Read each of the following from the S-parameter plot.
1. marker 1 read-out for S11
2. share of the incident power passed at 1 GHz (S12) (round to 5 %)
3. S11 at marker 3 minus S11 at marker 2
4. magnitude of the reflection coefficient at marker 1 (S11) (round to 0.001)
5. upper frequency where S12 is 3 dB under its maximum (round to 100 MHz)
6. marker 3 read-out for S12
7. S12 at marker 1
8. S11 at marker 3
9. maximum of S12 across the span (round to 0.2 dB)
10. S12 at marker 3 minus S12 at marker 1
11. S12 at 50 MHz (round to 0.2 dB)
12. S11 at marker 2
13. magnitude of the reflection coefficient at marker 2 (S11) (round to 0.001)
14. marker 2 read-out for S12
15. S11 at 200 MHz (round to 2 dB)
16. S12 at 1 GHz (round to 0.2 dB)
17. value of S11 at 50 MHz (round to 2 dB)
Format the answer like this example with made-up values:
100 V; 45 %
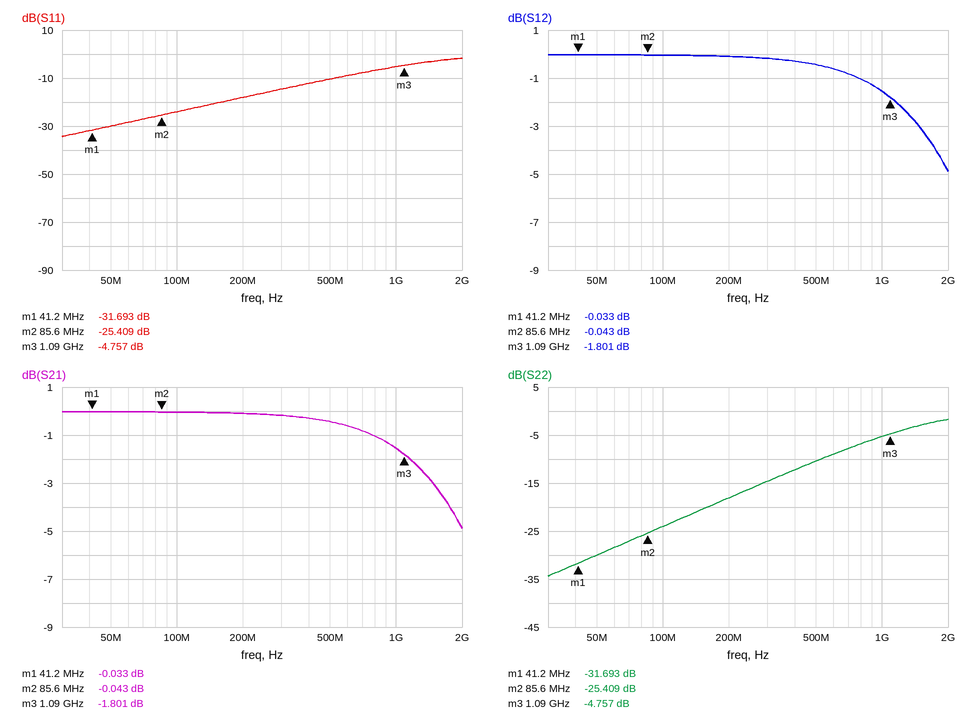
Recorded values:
-31.693 dB; 70 %; 20.652 dB; 0.026; 1.5 GHz; -1.801 dB; -0.033 dB; -4.757 dB; 0.0 dB; -1.768 dB; 0.0 dB; -25.409 dB; 0.054; -0.043 dB; -18 dB; -1.6 dB; -30 dB
